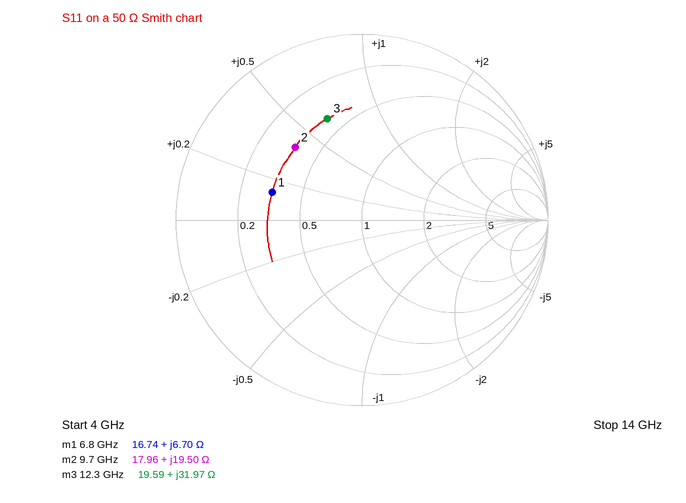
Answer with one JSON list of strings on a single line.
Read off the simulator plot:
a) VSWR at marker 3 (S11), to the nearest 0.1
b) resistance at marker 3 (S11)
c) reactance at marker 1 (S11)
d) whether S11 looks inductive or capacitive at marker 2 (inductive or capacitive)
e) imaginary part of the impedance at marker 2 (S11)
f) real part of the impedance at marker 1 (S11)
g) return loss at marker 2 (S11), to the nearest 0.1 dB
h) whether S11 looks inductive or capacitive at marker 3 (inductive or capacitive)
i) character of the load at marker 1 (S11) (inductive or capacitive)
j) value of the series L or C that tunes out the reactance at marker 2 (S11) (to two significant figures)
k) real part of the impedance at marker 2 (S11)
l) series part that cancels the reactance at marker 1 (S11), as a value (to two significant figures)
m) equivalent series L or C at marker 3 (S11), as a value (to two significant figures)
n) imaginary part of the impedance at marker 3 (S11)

["3.7", "19.59 Ω", "+6.70 Ω", "inductive", "+19.50 Ω", "16.74 Ω", "5.5 dB", "inductive", "inductive", "840 fF", "17.96 Ω", "3.5 pF", "410 pH", "+31.97 Ω"]
